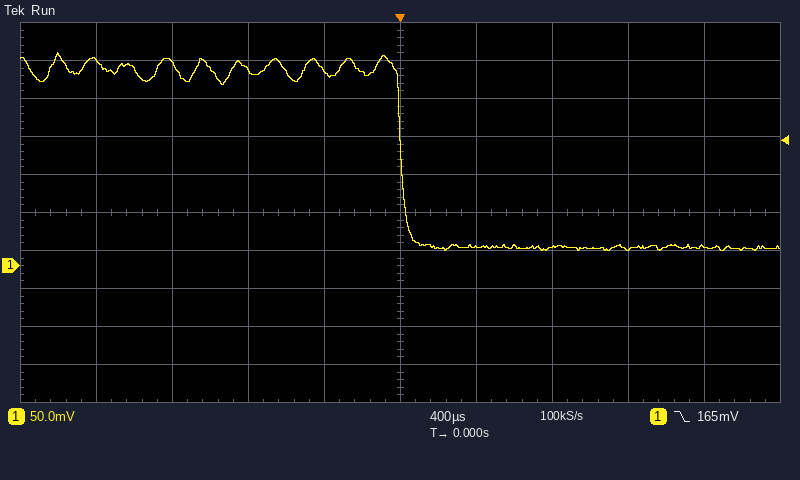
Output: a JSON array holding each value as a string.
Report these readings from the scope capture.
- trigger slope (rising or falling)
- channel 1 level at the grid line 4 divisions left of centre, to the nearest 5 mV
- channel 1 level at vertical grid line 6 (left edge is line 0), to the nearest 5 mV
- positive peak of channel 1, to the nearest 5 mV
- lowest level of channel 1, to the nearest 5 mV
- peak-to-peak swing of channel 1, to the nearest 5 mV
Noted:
["falling", "270 mV", "25 mV", "280 mV", "20 mV", "260 mV"]
